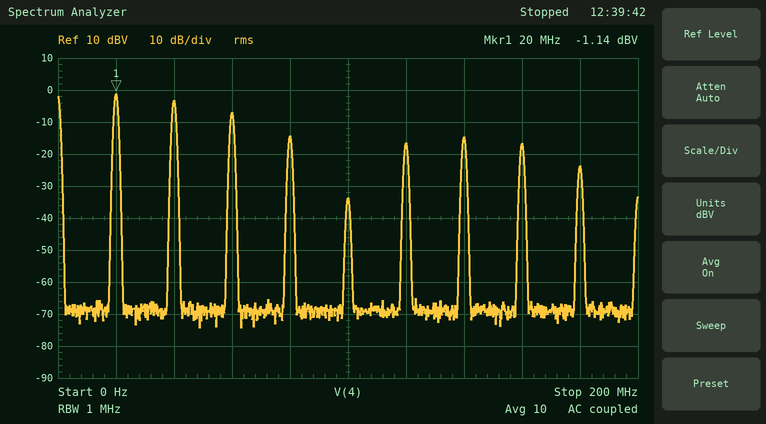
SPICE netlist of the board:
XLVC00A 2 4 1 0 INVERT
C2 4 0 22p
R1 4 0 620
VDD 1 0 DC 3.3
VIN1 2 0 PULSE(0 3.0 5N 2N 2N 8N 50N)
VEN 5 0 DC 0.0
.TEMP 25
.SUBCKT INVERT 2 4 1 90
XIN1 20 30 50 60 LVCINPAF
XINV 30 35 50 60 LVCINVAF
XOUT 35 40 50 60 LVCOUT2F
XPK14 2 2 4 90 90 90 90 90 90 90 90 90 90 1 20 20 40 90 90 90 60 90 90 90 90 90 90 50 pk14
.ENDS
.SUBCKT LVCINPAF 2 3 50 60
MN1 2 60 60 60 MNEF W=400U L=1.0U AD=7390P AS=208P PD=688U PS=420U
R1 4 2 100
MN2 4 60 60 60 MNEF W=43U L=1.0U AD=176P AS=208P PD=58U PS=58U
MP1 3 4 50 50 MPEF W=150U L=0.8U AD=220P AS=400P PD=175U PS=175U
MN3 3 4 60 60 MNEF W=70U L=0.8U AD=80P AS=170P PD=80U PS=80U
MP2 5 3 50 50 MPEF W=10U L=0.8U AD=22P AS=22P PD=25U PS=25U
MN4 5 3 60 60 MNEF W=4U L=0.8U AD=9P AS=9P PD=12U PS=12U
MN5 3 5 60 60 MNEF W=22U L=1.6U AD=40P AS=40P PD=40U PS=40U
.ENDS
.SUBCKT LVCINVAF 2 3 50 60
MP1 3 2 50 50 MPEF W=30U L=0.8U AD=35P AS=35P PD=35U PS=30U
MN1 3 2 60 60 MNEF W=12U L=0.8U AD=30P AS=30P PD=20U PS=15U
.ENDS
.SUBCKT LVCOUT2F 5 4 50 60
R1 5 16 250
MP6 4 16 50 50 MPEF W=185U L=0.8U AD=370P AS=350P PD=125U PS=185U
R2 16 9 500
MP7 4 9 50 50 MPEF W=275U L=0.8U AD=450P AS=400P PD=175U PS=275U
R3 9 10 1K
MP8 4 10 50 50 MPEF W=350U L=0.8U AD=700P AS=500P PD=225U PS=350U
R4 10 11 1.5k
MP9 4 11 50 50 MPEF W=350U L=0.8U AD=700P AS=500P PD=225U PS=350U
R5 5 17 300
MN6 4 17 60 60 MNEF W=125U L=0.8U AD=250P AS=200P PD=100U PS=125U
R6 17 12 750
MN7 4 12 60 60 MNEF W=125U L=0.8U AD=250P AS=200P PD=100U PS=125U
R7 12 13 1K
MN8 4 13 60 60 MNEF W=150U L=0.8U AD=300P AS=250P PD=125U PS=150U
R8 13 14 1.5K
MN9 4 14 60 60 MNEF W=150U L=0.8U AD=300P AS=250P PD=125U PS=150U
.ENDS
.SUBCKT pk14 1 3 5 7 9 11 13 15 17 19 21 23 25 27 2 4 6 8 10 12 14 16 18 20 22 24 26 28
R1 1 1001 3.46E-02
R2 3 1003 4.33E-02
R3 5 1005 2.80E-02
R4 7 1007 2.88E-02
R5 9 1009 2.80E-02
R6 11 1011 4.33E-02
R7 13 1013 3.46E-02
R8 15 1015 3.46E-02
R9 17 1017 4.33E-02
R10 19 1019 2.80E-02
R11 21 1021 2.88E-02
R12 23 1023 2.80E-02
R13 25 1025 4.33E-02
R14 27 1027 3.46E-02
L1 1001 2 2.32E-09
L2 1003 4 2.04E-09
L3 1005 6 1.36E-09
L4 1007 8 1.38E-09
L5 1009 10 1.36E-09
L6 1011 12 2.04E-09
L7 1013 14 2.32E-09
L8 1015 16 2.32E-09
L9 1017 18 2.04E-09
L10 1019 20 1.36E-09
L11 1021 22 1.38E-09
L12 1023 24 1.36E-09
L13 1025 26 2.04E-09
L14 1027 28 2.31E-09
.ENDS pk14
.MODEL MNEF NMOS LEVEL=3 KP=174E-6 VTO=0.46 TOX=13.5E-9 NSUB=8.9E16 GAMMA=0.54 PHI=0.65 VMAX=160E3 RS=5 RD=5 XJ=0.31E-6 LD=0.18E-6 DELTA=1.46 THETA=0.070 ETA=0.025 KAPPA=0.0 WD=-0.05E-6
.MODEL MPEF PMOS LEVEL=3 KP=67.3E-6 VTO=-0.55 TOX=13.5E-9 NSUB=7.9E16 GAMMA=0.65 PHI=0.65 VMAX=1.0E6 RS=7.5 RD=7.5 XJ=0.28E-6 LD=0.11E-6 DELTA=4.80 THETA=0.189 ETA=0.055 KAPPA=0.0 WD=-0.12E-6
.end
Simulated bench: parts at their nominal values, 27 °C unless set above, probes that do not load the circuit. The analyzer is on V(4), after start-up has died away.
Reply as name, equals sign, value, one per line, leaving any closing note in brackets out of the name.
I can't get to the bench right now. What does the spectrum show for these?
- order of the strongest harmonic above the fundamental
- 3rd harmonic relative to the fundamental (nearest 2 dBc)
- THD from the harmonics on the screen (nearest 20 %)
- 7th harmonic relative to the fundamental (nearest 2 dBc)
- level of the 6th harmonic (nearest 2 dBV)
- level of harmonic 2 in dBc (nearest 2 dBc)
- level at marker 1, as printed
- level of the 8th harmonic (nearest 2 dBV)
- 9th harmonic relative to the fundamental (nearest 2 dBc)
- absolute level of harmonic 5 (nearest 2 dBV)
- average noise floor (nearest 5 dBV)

order of the strongest harmonic above the fundamental = 2
3rd harmonic relative to the fundamental = -6 dBc
THD from the harmonics on the screen = 100 %
7th harmonic relative to the fundamental = -14 dBc
level of the 6th harmonic = -16 dBV
level of harmonic 2 in dBc = -2 dBc
level at marker 1, as printed = -1.14 dBV
level of the 8th harmonic = -16 dBV
9th harmonic relative to the fundamental = -22 dBc
absolute level of harmonic 5 = -34 dBV
average noise floor = -70 dBV
